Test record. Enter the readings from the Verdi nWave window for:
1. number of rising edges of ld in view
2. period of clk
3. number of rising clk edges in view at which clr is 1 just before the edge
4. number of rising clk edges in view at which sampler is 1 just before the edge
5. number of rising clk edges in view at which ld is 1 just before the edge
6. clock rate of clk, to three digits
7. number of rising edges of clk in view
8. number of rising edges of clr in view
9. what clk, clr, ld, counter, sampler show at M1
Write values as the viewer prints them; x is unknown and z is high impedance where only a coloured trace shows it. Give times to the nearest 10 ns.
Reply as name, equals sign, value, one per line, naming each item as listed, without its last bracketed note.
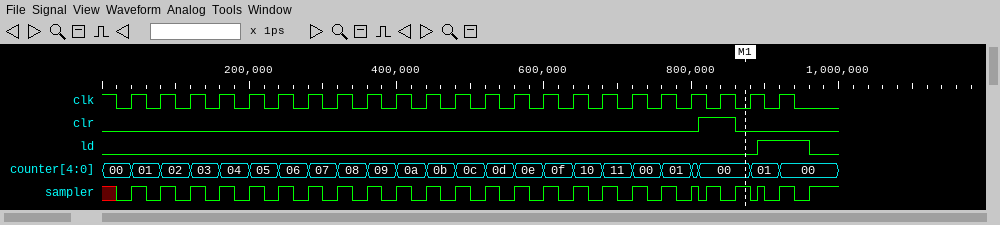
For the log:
number of rising edges of ld in view = 1
period of clk = 40 ns
number of rising clk edges in view at which clr is 1 just before the edge = 1
number of rising clk edges in view at which sampler is 1 just before the edge = 2
number of rising clk edges in view at which ld is 1 just before the edge = 1
clock rate of clk, to three digits = 25.0 MHz
number of rising edges of clk in view = 23
number of rising edges of clr in view = 1
what clk, clr, ld, counter, sampler show at M1 = clk=0, clr=0, ld=0, counter=00, sampler=1
